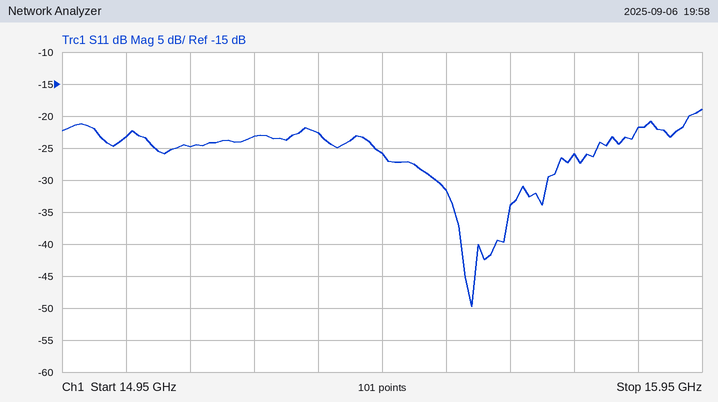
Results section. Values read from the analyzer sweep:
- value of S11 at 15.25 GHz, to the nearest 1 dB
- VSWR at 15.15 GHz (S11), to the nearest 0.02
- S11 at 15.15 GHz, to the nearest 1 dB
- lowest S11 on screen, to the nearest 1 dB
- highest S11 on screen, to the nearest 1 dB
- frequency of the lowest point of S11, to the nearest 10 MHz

-23 dB
1.12
-25 dB
-50 dB
-19 dB
15.59 GHz
